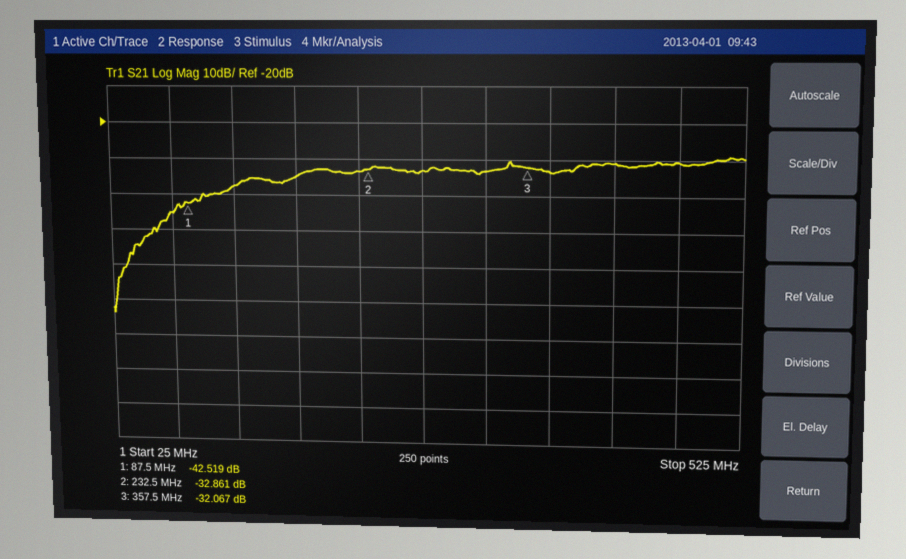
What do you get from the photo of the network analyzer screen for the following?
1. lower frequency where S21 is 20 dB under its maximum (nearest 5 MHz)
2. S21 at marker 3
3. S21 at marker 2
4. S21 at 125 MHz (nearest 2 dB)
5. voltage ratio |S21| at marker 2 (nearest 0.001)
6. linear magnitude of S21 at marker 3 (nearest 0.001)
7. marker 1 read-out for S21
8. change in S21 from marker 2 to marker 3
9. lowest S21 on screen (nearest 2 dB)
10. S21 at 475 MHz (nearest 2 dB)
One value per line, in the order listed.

65 MHz
-32.067 dB
-32.861 dB
-38 dB
0.023
0.025
-42.519 dB
0.794 dB
-74 dB
-30 dB
